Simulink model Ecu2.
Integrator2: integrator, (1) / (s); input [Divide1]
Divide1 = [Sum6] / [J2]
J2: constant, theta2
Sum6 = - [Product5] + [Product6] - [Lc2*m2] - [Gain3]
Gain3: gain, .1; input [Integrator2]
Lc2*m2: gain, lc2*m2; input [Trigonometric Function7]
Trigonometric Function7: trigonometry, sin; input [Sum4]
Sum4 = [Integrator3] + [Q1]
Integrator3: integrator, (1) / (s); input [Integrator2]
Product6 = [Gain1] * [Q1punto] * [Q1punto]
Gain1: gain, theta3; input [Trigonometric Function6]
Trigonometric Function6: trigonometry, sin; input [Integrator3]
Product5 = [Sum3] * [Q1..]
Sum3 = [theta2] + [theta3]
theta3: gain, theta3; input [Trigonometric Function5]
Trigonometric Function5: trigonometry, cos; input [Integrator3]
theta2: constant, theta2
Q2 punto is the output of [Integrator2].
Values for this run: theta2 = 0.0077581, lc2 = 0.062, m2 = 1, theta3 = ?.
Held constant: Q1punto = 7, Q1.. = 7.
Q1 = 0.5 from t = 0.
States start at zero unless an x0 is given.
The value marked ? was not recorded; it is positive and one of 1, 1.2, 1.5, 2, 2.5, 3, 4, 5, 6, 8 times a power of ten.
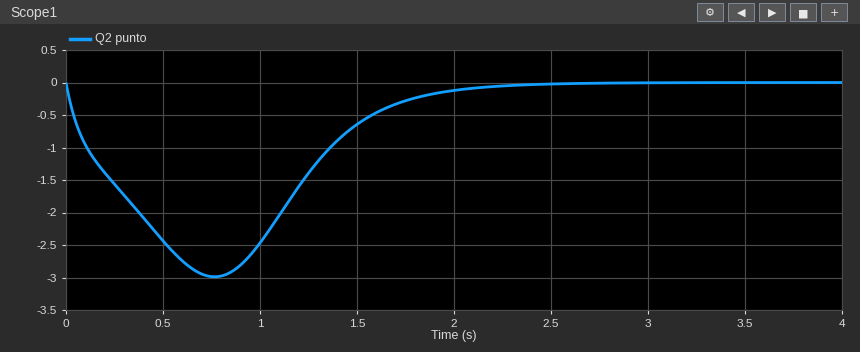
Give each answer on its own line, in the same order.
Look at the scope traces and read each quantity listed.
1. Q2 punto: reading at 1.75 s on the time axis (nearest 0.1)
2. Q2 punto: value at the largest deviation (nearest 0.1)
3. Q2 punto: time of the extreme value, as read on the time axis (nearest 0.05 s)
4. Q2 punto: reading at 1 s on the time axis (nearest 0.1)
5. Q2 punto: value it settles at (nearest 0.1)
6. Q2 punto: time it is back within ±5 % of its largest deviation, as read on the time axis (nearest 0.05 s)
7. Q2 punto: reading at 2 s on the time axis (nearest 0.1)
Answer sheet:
-0.3
-3.0
0.75 s
-2.5
0.0
1.95 s
-0.1
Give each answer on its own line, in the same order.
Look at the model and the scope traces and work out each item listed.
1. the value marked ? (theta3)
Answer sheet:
0.006
